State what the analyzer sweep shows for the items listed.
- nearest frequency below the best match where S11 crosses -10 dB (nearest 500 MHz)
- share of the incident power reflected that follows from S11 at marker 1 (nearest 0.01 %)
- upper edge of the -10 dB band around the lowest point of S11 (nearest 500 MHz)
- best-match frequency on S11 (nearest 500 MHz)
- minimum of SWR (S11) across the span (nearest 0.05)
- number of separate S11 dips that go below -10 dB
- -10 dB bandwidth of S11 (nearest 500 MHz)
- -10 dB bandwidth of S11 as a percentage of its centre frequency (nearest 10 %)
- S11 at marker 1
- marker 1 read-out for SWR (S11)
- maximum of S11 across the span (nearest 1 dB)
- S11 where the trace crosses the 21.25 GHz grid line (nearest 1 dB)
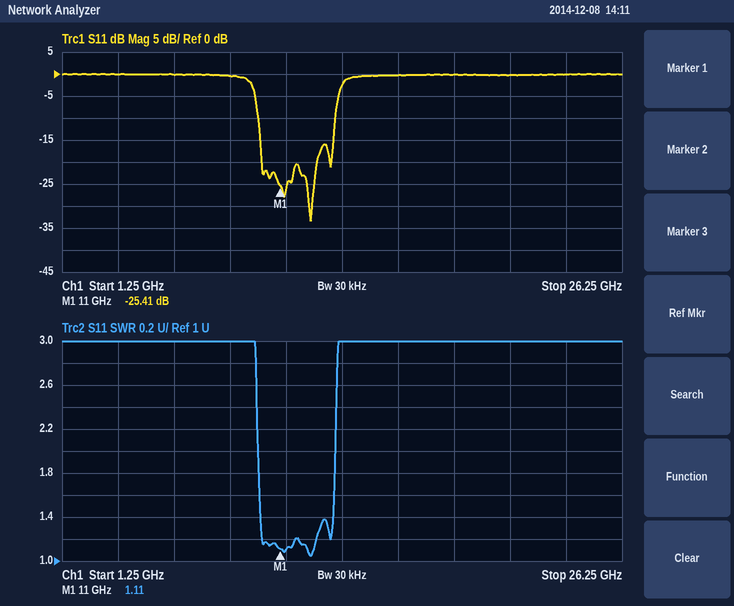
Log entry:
10.0 GHz
0.29 %
13.5 GHz
12.5 GHz
1.05
3
3.5 GHz
30 %
-25.41 dB
1.11
0 dB
0 dB
